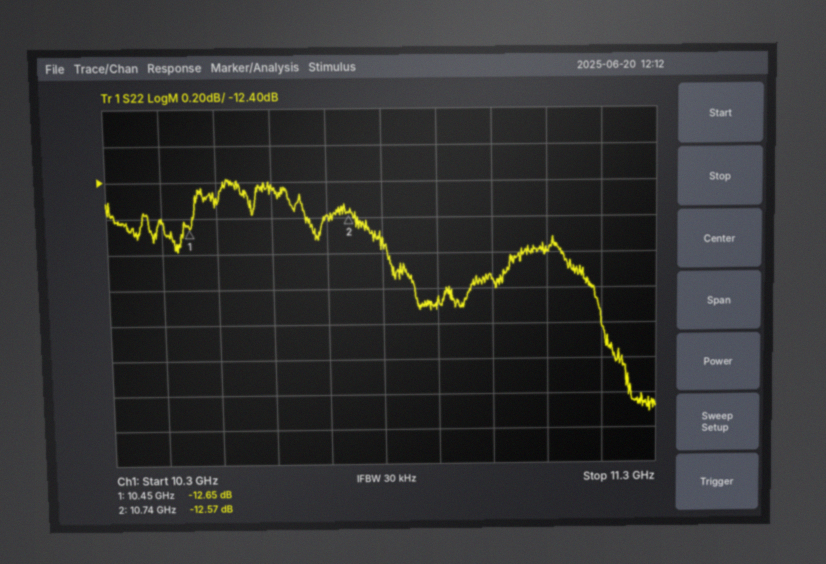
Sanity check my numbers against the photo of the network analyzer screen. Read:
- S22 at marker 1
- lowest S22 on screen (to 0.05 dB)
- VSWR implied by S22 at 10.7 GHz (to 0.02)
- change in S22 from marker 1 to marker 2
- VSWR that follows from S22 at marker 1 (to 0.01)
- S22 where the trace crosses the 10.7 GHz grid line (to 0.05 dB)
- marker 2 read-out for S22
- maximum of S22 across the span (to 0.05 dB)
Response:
-12.65 dB
-13.70 dB
1.62
0.08 dB
1.61
-12.60 dB
-12.57 dB
-12.40 dB
